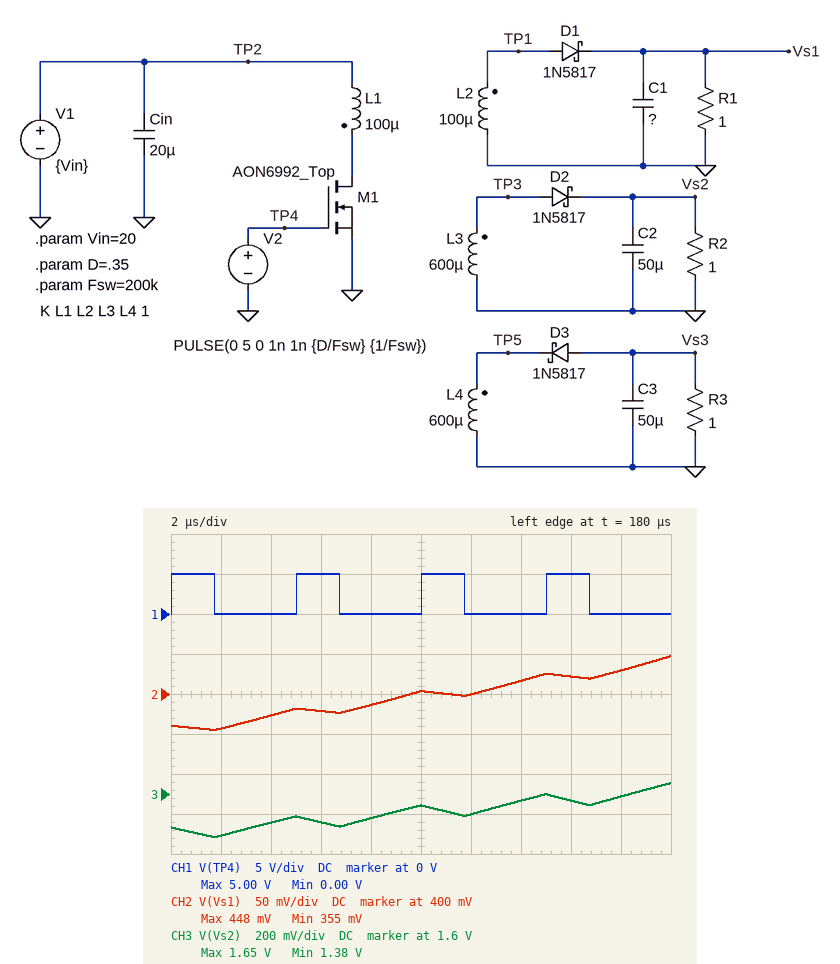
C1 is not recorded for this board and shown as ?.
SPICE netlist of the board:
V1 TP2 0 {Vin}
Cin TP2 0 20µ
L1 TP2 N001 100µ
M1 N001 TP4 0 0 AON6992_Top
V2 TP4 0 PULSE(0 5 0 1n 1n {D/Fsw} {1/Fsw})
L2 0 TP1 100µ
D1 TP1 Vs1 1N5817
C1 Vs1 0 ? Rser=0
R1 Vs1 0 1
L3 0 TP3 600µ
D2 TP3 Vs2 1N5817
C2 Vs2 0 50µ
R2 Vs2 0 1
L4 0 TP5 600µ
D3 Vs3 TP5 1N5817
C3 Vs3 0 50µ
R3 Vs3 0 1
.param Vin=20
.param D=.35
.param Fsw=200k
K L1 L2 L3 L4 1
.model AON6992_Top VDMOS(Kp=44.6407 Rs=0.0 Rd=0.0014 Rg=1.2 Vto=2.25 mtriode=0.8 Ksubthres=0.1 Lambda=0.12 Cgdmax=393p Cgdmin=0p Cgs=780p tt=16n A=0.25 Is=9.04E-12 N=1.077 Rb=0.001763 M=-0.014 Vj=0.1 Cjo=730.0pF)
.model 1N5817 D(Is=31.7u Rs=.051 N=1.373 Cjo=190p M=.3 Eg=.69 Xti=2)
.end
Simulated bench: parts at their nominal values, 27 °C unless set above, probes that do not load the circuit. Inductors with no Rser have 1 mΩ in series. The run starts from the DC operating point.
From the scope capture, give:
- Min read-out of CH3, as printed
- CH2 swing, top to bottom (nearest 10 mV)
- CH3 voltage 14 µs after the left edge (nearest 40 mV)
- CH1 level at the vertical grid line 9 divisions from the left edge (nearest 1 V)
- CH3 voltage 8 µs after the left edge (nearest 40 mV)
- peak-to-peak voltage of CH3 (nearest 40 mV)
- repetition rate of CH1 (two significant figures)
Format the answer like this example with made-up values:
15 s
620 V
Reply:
1.38 V
90 mV
1.56 V
0 V
1.48 V
280 mV
200 kHz
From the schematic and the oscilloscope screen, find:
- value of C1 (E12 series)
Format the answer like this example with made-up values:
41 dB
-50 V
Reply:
120 µF
